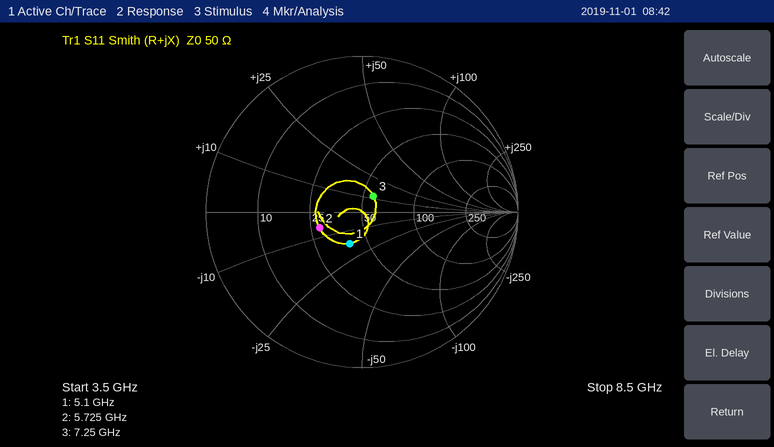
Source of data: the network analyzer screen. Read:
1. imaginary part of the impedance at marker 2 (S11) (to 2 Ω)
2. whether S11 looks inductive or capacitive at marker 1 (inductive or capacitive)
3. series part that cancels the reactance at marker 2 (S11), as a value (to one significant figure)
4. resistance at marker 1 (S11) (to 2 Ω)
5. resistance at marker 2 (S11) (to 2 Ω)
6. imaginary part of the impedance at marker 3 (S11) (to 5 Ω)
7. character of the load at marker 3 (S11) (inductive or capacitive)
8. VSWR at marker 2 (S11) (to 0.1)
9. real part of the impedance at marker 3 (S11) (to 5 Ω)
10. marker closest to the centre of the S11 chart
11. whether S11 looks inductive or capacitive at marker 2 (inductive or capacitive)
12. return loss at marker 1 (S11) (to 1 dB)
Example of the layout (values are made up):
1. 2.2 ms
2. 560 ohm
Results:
1. -6 Ω
2. capacitive
3. 200 pH
4. 40 Ω
5. 28 Ω
6. +10 Ω
7. inductive
8. 1.8
9. 55 Ω
10. marker 3
11. capacitive
12. 13 dB
